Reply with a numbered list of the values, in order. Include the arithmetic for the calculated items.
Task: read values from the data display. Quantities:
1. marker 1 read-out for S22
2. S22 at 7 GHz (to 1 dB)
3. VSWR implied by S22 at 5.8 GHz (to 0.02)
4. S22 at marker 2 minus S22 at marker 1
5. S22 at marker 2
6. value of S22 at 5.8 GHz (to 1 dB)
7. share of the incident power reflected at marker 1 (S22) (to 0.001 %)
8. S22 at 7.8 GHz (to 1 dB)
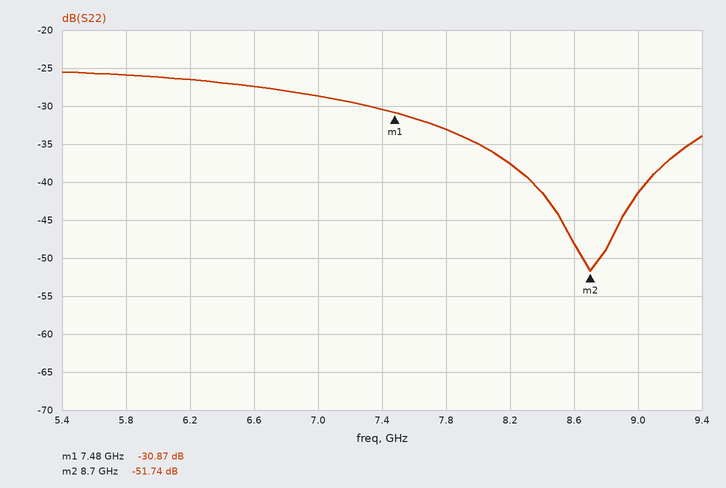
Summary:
1. -30.87 dB
2. -29 dB
3. |Γ| = 10^(-26/20) = 0.0501; VSWR = (1 + 0.0501)/(1 − 0.0501) ≈ 1.11, so 1.10 to the nearest 0.02
4. -51.74 − (-30.87) = -20.87 dB
5. -51.74 dB
6. -26 dB
7. 10^(-30.87/10) ≈ 0.082 %
8. -33 dB
